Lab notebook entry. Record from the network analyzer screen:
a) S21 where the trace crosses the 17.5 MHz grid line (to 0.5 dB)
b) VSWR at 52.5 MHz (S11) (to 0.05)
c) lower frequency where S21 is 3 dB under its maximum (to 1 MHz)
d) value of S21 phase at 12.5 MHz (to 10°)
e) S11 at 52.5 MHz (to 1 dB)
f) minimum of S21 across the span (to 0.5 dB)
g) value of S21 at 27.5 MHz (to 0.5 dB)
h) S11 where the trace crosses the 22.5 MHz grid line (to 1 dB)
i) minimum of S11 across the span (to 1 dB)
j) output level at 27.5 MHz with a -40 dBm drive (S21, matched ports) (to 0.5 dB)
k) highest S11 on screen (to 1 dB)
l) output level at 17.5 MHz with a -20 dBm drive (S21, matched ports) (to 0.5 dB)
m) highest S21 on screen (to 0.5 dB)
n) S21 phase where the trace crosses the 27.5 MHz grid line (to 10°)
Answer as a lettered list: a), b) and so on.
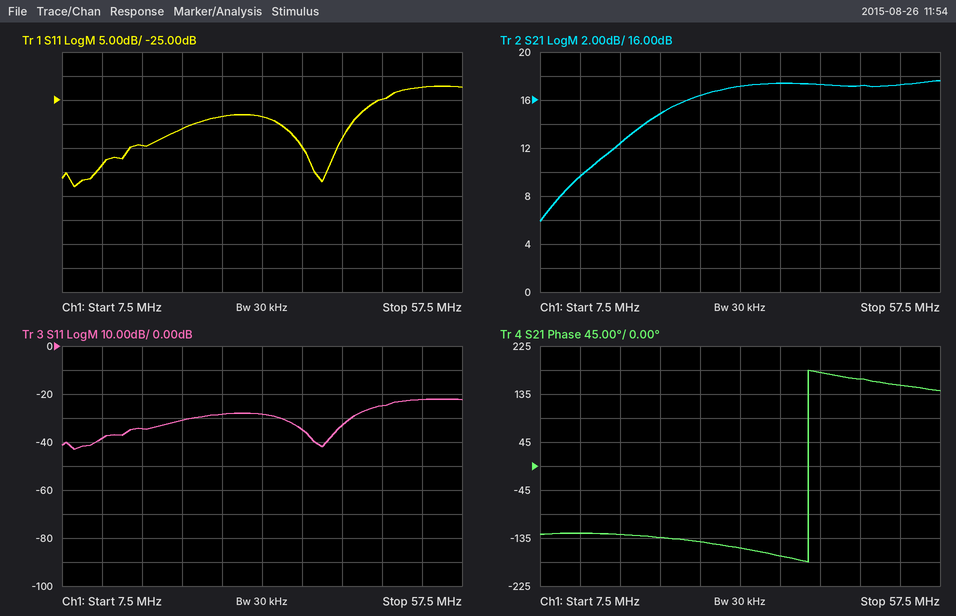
a) 12.5 dB
b) 1.15
c) 22 MHz
d) -130°
e) -22 dB
f) 6.0 dB
g) 16.5 dB
h) -31 dB
i) -43 dB
j) -23.5 dBm
k) -22 dB
l) -7.5 dBm
m) 17.5 dB
n) -140°
